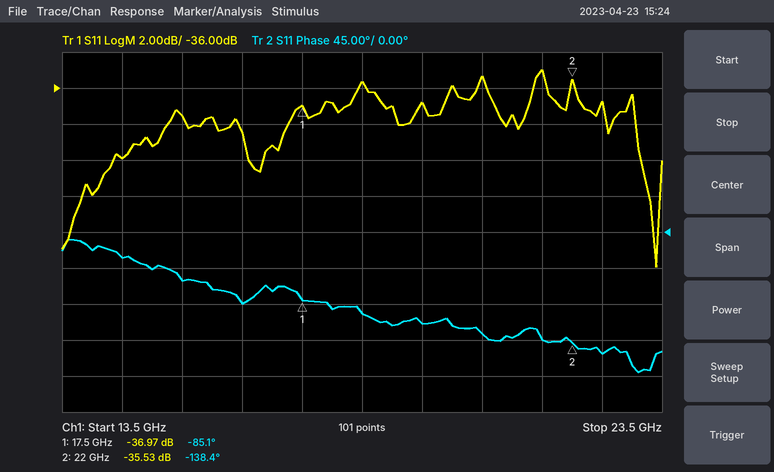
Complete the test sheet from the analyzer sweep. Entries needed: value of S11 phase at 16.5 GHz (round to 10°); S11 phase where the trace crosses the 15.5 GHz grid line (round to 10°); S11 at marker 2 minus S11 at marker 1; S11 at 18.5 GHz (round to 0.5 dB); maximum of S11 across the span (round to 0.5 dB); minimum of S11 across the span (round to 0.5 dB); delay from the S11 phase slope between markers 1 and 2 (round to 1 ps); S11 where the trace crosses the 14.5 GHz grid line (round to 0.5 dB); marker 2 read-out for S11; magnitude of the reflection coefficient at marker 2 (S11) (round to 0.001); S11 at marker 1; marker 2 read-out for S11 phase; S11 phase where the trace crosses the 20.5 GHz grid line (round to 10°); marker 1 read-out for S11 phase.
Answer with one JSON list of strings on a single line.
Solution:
["-90°", "-60°", "1.44 dB", "-35.5 dB", "-35.0 dB", "-46.0 dB", "33 ps", "-40.0 dB", "-35.53 dB", "0.017", "-36.97 dB", "-138.4°", "-130°", "-85.1°"]
